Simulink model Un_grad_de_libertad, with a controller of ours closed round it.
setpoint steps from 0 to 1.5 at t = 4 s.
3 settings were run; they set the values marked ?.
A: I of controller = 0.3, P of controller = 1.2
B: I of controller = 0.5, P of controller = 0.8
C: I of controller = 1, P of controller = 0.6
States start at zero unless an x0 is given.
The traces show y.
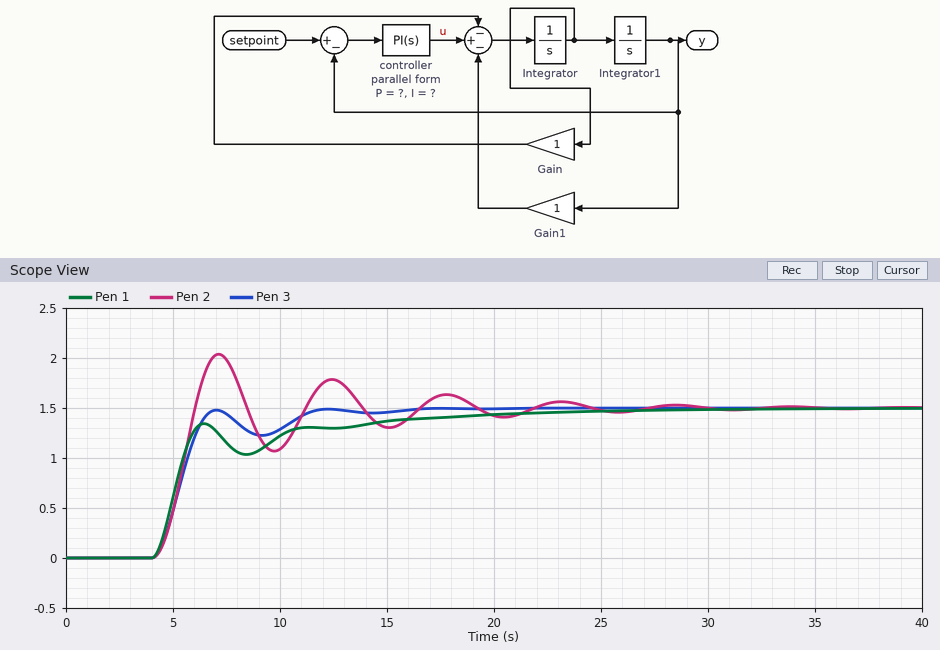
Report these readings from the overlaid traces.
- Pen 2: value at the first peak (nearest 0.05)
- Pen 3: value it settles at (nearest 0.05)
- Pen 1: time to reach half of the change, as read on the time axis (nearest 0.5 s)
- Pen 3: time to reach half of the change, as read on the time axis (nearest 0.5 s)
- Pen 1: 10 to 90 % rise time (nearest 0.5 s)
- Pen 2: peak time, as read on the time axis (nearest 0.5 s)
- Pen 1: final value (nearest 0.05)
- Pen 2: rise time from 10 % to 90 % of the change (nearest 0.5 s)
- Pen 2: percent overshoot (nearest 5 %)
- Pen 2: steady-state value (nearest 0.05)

2.05
1.50
5.0 s
5.5 s
10.0 s
7.0 s
1.50
1.5 s
35 %
1.50
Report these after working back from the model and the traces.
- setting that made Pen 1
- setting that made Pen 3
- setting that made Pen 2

A
B
C
